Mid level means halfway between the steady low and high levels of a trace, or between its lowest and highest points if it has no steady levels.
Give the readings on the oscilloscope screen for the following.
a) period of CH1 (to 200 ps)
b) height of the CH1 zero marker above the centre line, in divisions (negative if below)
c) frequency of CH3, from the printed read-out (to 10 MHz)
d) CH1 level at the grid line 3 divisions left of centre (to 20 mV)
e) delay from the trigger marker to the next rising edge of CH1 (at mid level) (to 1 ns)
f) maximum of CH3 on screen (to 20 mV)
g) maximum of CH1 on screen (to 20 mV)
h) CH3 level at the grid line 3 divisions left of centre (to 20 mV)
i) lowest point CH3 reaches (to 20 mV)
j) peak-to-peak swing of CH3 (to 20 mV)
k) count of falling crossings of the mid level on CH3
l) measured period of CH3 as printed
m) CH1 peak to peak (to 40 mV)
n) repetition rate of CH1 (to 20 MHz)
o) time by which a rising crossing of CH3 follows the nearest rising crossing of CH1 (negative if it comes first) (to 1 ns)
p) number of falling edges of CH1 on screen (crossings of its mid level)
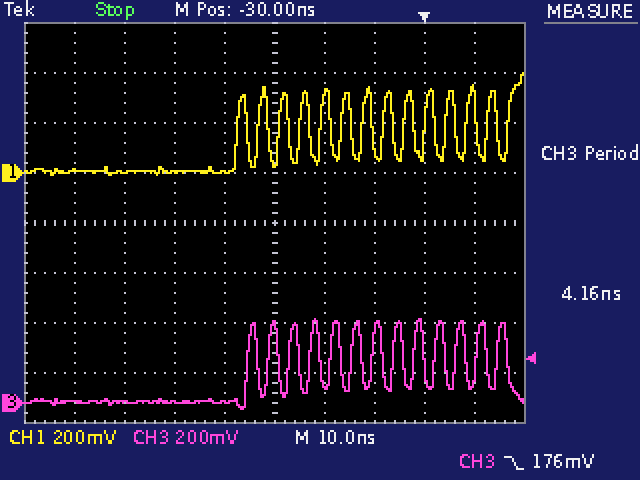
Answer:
4.2 ns
+1.0 div
240 MHz
0 mV
4 ns
340 mV
400 mV
0 mV
-20 mV
360 mV
13
4.16 ns
400 mV
240 MHz
+2 ns
13
